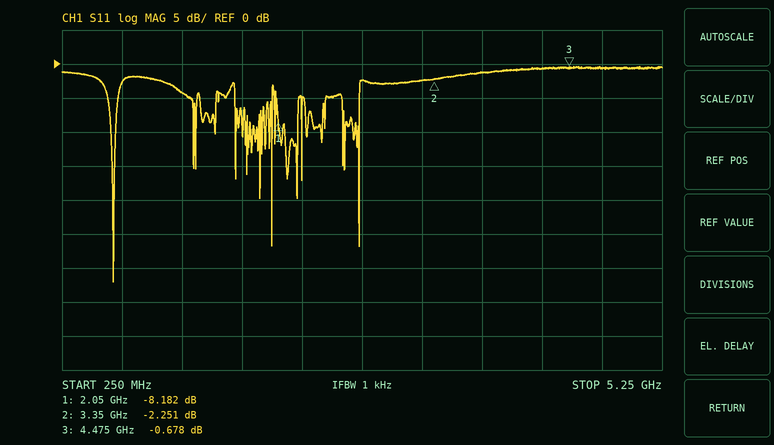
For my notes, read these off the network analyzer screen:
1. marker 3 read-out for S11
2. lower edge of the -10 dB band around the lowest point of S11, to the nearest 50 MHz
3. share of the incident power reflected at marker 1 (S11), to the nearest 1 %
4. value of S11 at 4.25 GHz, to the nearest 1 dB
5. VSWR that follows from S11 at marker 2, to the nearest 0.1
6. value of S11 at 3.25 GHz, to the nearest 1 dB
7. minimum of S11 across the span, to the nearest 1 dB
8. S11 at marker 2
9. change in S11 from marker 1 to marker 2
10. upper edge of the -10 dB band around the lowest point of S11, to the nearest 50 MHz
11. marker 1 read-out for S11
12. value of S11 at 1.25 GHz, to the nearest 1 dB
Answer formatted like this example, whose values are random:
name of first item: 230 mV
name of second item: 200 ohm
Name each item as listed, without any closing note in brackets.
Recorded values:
marker 3 read-out for S11: -0.678 dB
lower edge of the -10 dB band around the lowest point of S11, to the nearest 50 MHz: 650 MHz
share of the incident power reflected at marker 1 (S11), to the nearest 1 %: 15 %
value of S11 at 4.25 GHz, to the nearest 1 dB: -1 dB
VSWR that follows from S11 at marker 2, to the nearest 0.1: 7.8
value of S11 at 3.25 GHz, to the nearest 1 dB: -2 dB
minimum of S11 across the span, to the nearest 1 dB: -32 dB
S11 at marker 2: -2.251 dB
change in S11 from marker 1 to marker 2: 5.931 dB
upper edge of the -10 dB band around the lowest point of S11, to the nearest 50 MHz: 700 MHz
marker 1 read-out for S11: -8.182 dB
value of S11 at 1.25 GHz, to the nearest 1 dB: -4 dB
